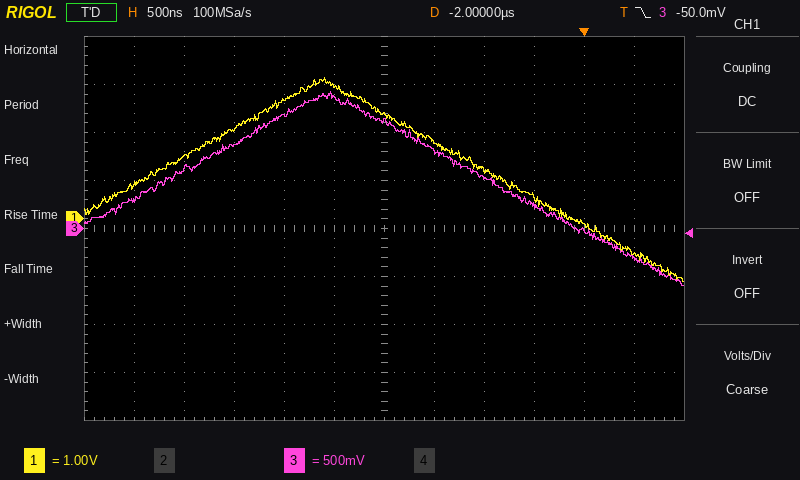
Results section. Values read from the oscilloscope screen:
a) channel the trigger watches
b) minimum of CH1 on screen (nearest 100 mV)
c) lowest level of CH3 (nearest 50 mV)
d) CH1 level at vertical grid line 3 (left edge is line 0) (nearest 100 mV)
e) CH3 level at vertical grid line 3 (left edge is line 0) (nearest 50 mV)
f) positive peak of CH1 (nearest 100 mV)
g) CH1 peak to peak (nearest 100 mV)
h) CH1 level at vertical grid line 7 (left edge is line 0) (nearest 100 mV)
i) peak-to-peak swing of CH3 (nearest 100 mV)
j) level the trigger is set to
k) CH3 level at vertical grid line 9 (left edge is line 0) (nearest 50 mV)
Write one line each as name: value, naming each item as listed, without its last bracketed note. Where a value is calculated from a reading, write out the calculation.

channel the trigger watches: CH3
minimum of CH1 on screen: -1.3 V
lowest level of CH3: -600 mV
CH1 level at vertical grid line 3 (left edge is line 0): 1.9 V
CH3 level at vertical grid line 3 (left edge is line 0): 850 mV
positive peak of CH1: 2.9 V
CH1 peak to peak: 2.9 V − (-1.3 V) = 4.2 V
CH1 level at vertical grid line 7 (left edge is line 0): 1.6 V
peak-to-peak swing of CH3: 2.00 V
level the trigger is set to: -50.0 mV
CH3 level at vertical grid line 9 (left edge is line 0): 250 mV
